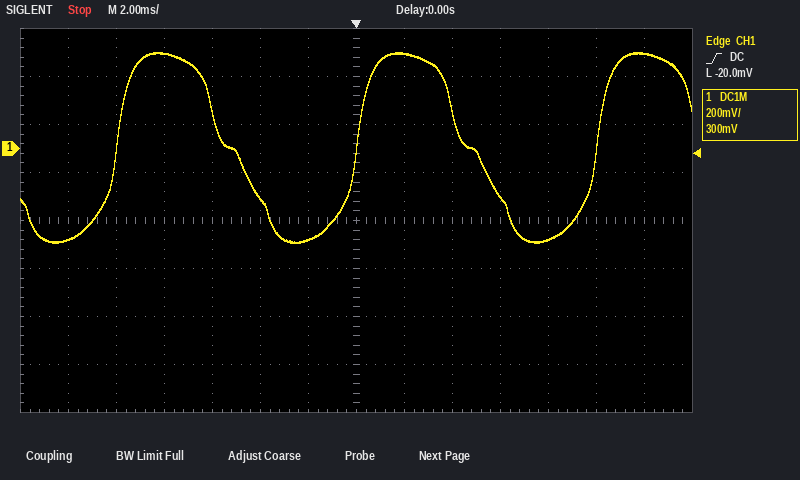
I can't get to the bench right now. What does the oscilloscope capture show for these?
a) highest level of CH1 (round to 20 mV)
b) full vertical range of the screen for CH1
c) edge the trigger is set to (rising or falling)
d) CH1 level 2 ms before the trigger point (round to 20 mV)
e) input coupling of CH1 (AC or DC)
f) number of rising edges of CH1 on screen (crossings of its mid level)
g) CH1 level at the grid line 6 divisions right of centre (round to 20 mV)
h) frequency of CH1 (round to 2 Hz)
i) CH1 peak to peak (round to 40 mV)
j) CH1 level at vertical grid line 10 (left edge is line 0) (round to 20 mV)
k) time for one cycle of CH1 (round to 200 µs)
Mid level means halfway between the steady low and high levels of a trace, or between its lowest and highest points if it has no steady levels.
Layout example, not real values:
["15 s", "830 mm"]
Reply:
["400 mV", "1.6 V", "rising", "-380 mV", "DC", "3", "400 mV", "100 Hz", "800 mV", "-200 mV", "10.0 ms"]
